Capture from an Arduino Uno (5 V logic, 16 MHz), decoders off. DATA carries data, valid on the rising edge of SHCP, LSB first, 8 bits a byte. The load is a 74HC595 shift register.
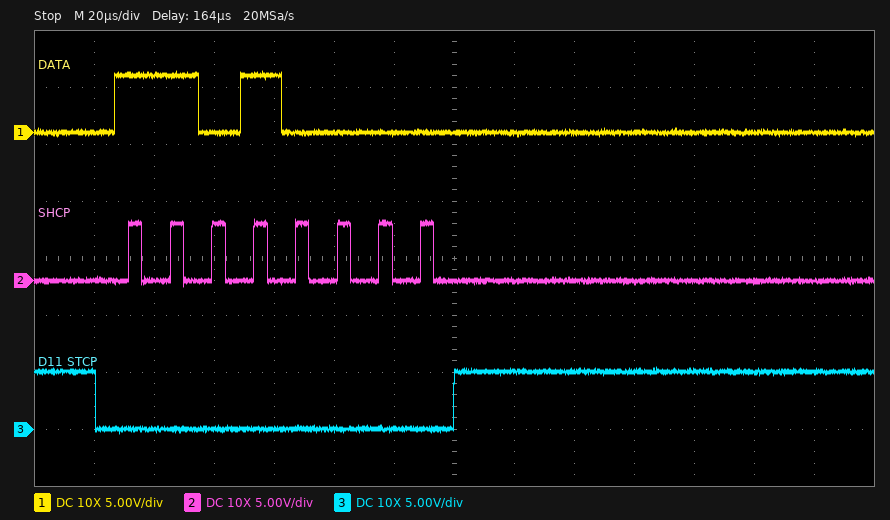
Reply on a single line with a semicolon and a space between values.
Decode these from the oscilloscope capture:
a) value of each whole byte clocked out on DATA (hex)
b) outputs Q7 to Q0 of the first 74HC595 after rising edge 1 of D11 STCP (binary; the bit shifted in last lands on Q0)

0x0B; 11010000
